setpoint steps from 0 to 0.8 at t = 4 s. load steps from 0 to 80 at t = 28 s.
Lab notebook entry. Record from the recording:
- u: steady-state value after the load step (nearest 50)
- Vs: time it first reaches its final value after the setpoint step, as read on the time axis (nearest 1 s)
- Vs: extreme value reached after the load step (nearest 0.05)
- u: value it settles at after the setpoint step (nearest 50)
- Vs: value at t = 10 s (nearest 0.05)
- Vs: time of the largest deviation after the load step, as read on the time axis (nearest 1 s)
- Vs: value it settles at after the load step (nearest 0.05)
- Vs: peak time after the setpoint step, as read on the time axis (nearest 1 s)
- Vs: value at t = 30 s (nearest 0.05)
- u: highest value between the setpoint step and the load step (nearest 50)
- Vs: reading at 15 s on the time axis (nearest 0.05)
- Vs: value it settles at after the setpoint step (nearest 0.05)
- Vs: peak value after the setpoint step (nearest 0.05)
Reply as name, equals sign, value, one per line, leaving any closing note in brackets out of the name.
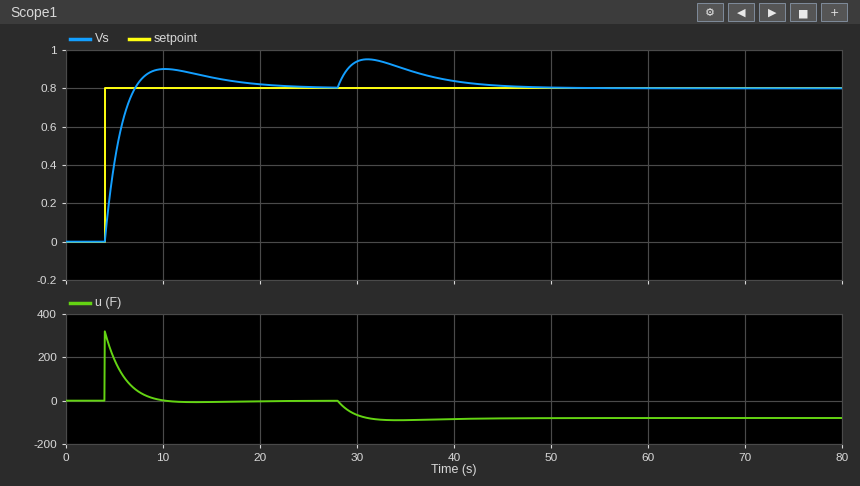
u: steady-state value after the load step = -100
Vs: time it first reaches its final value after the setpoint step, as read on the time axis = 7 s
Vs: extreme value reached after the load step = 0.95
u: value it settles at after the setpoint step = 0
Vs: value at t = 10 s = 0.90
Vs: time of the largest deviation after the load step, as read on the time axis = 31 s
Vs: value it settles at after the load step = 0.80
Vs: peak time after the setpoint step, as read on the time axis = 10 s
Vs: value at t = 30 s = 0.95
u: highest value between the setpoint step and the load step = 300
Vs: reading at 15 s on the time axis = 0.85
Vs: value it settles at after the setpoint step = 0.80
Vs: peak value after the setpoint step = 0.90
